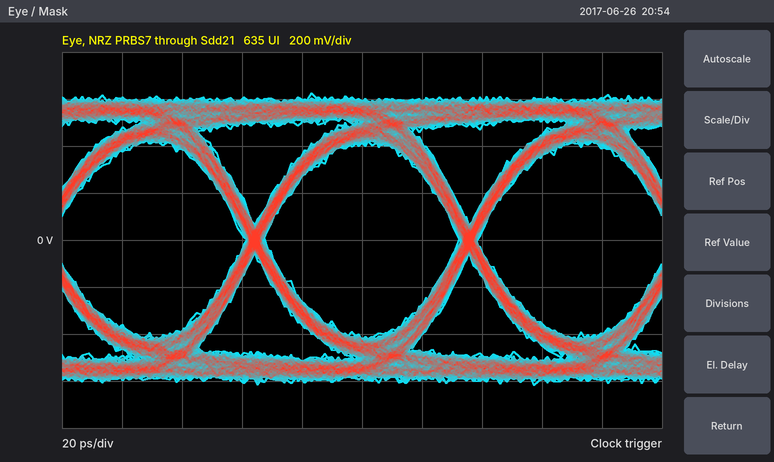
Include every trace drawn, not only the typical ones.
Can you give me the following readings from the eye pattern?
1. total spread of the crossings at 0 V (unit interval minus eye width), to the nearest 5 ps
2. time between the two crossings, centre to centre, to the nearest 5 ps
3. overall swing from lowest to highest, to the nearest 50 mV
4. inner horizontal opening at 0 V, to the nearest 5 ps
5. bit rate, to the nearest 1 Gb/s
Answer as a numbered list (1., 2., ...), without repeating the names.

1. 5 ps
2. 70 ps
3. 1.25 V
4. 65 ps
5. 14 Gb/s
